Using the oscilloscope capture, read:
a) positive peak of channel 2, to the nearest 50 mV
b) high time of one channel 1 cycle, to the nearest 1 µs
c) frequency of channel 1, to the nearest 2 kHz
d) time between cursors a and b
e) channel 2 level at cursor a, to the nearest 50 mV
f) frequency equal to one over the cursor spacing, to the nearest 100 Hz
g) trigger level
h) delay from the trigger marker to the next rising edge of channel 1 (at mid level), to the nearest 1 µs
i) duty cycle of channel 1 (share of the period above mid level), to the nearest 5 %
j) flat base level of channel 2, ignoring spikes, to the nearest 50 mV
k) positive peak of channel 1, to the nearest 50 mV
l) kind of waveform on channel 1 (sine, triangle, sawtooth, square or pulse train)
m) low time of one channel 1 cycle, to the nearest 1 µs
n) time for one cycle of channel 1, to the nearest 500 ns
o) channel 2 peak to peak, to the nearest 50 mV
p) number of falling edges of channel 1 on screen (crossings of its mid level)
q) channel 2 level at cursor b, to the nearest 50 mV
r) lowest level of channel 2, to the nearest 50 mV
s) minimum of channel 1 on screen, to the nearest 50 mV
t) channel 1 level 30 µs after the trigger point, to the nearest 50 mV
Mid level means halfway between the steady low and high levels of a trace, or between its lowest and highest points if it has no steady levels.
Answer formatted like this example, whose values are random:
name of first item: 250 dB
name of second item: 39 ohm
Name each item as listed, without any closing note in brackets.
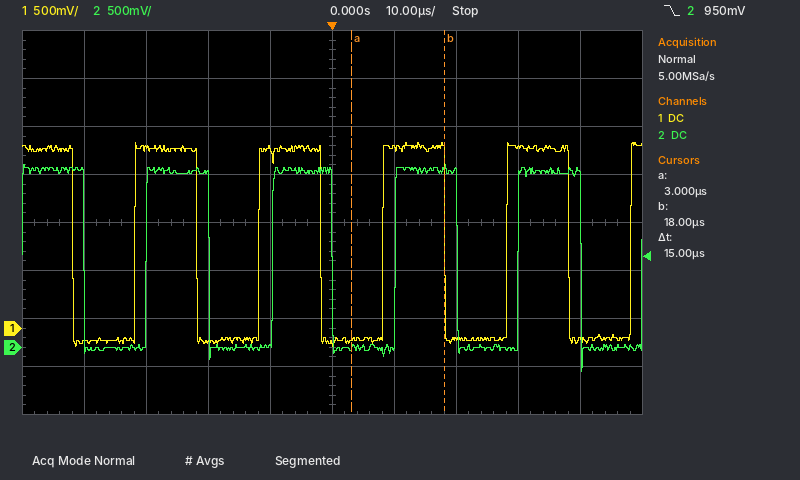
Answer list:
positive peak of channel 2, to the nearest 50 mV: 1.90 V
high time of one channel 1 cycle, to the nearest 1 µs: 10 µs
frequency of channel 1, to the nearest 2 kHz: 50 kHz
time between cursors a and b: 15 µs
channel 2 level at cursor a, to the nearest 50 mV: 0 mV
frequency equal to one over the cursor spacing, to the nearest 100 Hz: 66.7 kHz
trigger level: 950 mV
delay from the trigger marker to the next rising edge of channel 1 (at mid level), to the nearest 1 µs: 8 µs
duty cycle of channel 1 (share of the period above mid level), to the nearest 5 %: 50 %
flat base level of channel 2, ignoring spikes, to the nearest 50 mV: 0 mV
positive peak of channel 1, to the nearest 50 mV: 1.95 V
kind of waveform on channel 1: square
low time of one channel 1 cycle, to the nearest 1 µs: 10 µs
time for one cycle of channel 1, to the nearest 500 ns: 20.0 µs
channel 2 peak to peak, to the nearest 50 mV: 2.15 V
number of falling edges of channel 1 on screen: 5
channel 2 level at cursor b, to the nearest 50 mV: 1.85 V
lowest level of channel 2, to the nearest 50 mV: -250 mV
minimum of channel 1 on screen, to the nearest 50 mV: -200 mV
channel 1 level 30 µs after the trigger point, to the nearest 50 mV: 1.90 V
